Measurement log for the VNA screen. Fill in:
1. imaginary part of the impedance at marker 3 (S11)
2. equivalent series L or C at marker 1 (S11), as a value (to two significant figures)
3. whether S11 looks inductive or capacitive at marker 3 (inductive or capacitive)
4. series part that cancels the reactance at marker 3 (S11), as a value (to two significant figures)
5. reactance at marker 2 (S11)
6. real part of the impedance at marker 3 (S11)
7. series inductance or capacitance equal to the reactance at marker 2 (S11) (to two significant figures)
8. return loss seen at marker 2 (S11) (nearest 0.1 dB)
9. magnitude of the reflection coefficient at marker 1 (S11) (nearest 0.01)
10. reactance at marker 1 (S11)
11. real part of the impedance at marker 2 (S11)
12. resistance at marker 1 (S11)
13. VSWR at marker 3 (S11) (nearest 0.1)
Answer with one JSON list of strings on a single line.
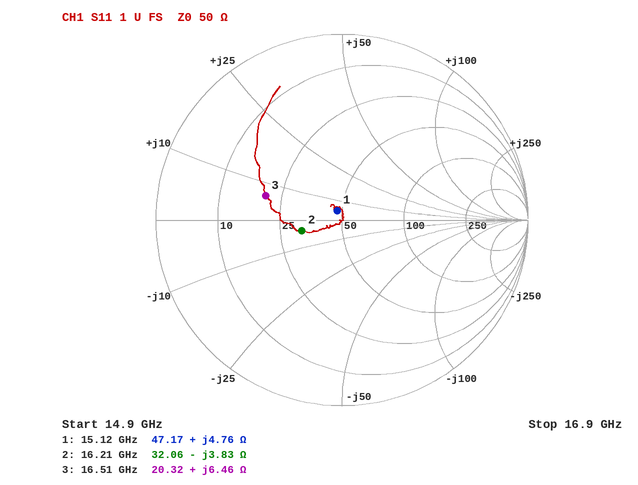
["+6.46 Ω", "50 pH", "inductive", "1.5 pF", "-3.83 Ω", "20.32 Ω", "2.6 pF", "13.0 dB", "0.06", "+4.76 Ω", "32.06 Ω", "47.17 Ω", "2.5"]
